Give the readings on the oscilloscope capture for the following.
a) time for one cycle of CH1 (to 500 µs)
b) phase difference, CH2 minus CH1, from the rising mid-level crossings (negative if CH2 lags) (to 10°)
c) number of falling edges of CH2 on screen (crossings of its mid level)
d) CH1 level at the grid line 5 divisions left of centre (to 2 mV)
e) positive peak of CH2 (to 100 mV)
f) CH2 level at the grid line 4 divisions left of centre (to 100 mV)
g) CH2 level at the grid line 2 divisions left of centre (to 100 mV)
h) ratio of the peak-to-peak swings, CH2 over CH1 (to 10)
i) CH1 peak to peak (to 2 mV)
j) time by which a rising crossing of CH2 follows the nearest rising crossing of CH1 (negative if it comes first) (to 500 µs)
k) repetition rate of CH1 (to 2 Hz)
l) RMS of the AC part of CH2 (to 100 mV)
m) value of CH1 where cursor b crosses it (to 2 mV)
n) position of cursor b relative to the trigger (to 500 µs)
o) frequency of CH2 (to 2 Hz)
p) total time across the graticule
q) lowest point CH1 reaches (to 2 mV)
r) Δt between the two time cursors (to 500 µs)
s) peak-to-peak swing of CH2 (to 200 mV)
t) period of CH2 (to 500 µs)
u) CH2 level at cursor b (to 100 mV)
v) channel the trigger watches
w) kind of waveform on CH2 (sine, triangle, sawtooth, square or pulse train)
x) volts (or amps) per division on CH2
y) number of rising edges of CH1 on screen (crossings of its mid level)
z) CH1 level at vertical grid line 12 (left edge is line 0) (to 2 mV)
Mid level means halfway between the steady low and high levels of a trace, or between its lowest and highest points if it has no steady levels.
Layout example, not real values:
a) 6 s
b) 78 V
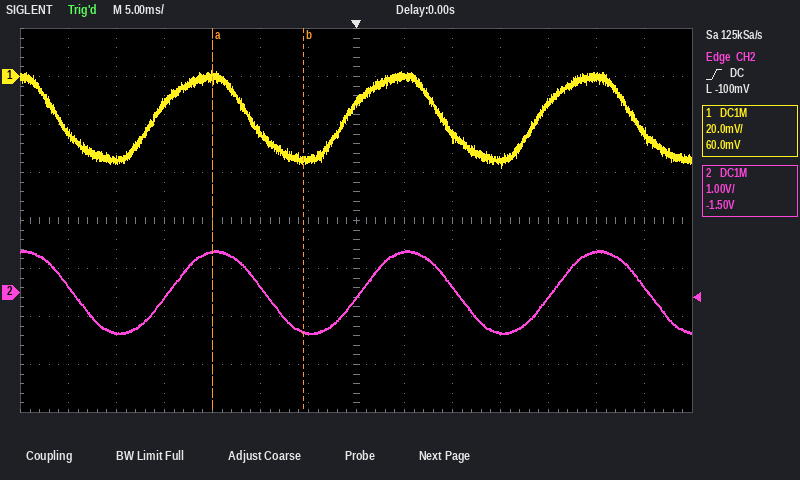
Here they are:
a) 20.0 ms
b) -30°
c) 4
d) -34 mV
e) 900 mV
f) -100 mV
g) 100 mV
h) 40
i) 40 mV
j) +1.5 ms
k) 50 Hz
l) 600 mV
m) -34 mV
n) -5.5 ms
o) 50 Hz
p) 70 ms
q) -38 mV
r) 9.5 ms
s) 1.8 V
t) 20.0 ms
u) -800 mV
v) CH2
w) sine
x) 1 V
y) 3
z) 0 mV
